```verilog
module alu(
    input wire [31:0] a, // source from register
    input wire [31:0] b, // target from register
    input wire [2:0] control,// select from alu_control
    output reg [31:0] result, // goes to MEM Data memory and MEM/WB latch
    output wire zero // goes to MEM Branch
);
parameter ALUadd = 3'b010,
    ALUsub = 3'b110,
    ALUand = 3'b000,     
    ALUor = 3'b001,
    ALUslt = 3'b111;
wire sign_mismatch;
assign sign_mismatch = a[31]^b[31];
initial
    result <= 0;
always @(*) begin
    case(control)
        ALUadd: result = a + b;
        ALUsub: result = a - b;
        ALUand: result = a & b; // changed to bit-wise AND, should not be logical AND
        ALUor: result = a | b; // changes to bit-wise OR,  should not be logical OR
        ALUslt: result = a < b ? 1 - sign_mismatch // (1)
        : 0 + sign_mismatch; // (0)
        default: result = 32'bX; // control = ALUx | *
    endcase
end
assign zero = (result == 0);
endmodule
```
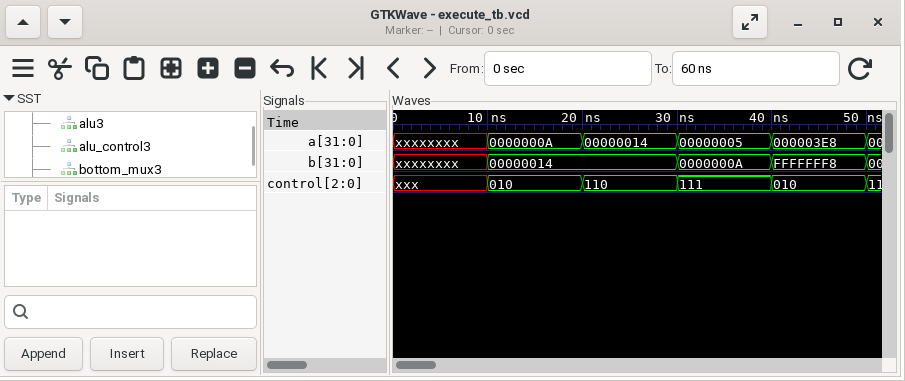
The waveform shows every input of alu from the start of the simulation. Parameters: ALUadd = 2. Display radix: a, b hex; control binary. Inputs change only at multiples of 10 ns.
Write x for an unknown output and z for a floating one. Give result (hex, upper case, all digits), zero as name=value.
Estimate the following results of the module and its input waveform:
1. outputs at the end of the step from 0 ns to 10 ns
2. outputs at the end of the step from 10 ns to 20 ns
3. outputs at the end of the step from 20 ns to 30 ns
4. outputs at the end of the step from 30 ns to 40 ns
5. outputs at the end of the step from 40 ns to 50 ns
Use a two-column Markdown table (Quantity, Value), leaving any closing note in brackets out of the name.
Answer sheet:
| Quantity | Value |
|---|---|
| outputs at the end of the step from 0 ns to 10 ns | result=00000000, zero=1 |
| outputs at the end of the step from 10 ns to 20 ns | result=0000001E, zero=0 |
| outputs at the end of the step from 20 ns to 30 ns | result=00000000, zero=1 |
| outputs at the end of the step from 30 ns to 40 ns | result=00000001, zero=0 |
| outputs at the end of the step from 40 ns to 50 ns | result=000003E0, zero=0 |
